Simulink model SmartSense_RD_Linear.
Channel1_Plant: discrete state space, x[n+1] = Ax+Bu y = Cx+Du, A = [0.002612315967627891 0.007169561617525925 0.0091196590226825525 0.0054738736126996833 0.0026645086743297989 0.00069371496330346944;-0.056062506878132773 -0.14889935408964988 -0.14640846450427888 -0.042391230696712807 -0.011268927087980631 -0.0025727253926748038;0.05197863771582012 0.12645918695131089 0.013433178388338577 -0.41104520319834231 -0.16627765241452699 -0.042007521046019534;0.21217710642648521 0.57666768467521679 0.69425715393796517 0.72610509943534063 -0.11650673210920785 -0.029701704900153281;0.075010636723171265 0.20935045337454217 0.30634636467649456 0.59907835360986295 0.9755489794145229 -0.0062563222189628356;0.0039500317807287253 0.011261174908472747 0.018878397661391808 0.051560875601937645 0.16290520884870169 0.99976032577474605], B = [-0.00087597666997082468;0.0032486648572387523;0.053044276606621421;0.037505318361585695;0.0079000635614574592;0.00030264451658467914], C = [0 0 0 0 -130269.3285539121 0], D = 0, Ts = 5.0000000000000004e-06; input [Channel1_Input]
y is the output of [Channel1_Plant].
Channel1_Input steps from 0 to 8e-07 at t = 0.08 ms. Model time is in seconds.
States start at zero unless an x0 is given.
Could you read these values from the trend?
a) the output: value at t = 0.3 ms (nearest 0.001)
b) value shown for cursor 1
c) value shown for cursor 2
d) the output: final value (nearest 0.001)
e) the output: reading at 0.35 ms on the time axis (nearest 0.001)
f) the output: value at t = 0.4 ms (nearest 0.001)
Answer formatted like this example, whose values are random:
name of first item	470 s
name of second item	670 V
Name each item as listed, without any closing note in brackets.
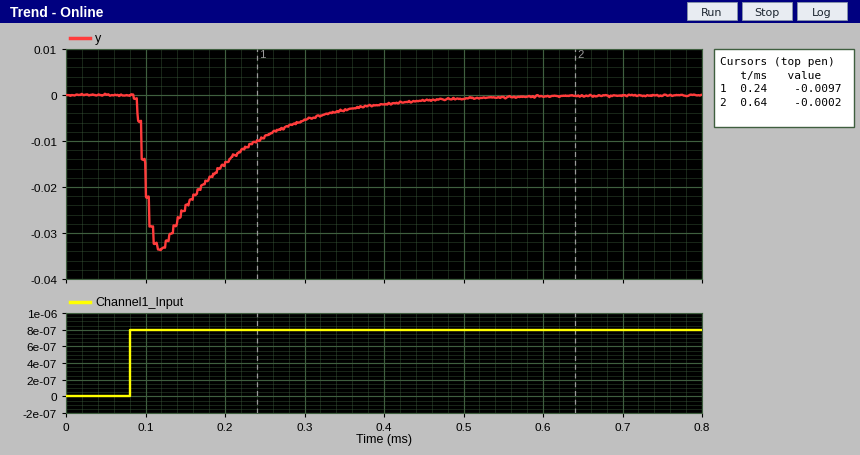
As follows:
the output: value at t = 0.3 ms	-0.005
value shown for cursor 1	-0.0097
value shown for cursor 2	-0.0002
the output: final value	0.000
the output: reading at 0.35 ms on the time axis	-0.003
the output: value at t = 0.4 ms	-0.002
